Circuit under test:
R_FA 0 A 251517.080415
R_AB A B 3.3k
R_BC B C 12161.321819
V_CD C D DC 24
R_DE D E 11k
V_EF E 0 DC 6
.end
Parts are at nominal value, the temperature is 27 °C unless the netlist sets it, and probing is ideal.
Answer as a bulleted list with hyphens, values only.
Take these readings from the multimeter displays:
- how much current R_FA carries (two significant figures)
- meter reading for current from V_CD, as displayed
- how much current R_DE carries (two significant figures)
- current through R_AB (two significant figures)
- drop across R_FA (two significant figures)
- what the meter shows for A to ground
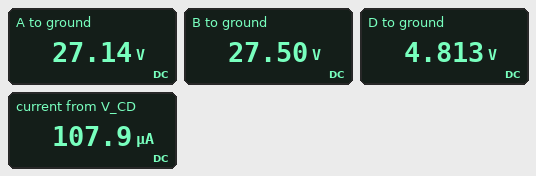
- 110 µA
- 107.9 µA
- 110 µA
- 110 µA
- 27 V
- 27.14 V
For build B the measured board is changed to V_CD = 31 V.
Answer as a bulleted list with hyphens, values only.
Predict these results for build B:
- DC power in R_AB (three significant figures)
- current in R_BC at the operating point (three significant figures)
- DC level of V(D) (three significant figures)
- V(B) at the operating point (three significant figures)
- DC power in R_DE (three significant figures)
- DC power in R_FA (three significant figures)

- 58.5 µW
- 133 µA
- 4.54 V
- 33.9 V
- 195 µW
- 4.46 mW
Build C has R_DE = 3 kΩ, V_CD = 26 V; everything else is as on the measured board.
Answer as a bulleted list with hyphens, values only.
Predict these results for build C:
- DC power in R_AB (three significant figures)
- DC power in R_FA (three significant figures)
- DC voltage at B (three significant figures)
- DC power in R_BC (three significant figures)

- 46.4 µW
- 3.53 mW
- 30.2 V
- 171 µW
